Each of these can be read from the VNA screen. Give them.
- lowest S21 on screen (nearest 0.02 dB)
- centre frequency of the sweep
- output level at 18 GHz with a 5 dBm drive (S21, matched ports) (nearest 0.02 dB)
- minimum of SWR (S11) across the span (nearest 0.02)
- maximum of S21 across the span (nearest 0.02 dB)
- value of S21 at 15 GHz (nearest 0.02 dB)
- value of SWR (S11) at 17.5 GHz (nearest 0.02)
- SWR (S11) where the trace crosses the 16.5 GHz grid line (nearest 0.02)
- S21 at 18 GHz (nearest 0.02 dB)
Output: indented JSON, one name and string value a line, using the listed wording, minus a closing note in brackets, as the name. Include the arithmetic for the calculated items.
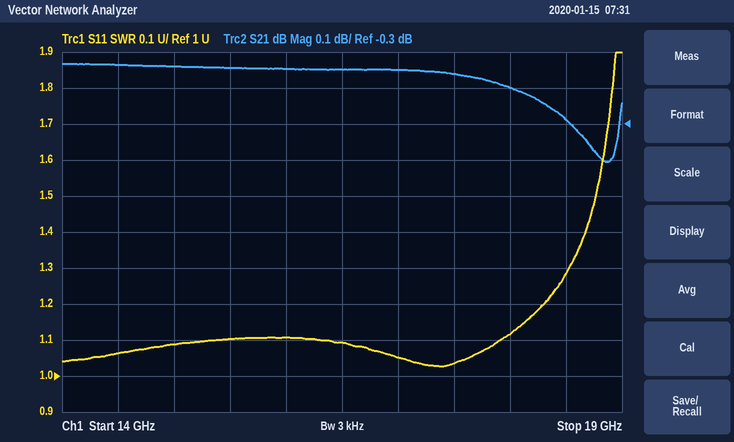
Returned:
{
  "lowest S21 on screen": "-0.40 dB",
  "centre frequency of the sweep": "16.5 GHz",
  "output level at 18 GHz with a 5 dBm drive (S21, matched ports)": "5 dBm + (-0.20 dB) = 4.80 dBm",
  "minimum of SWR (S11) across the span": "1.02",
  "maximum of S21 across the span": "-0.14 dB",
  "value of S21 at 15 GHz": "-0.14 dB",
  "value of SWR (S11) at 17.5 GHz": "1.04",
  "SWR (S11) where the trace crosses the 16.5 GHz grid line": "1.10",
  "S21 at 18 GHz": "-0.20 dB"
}
